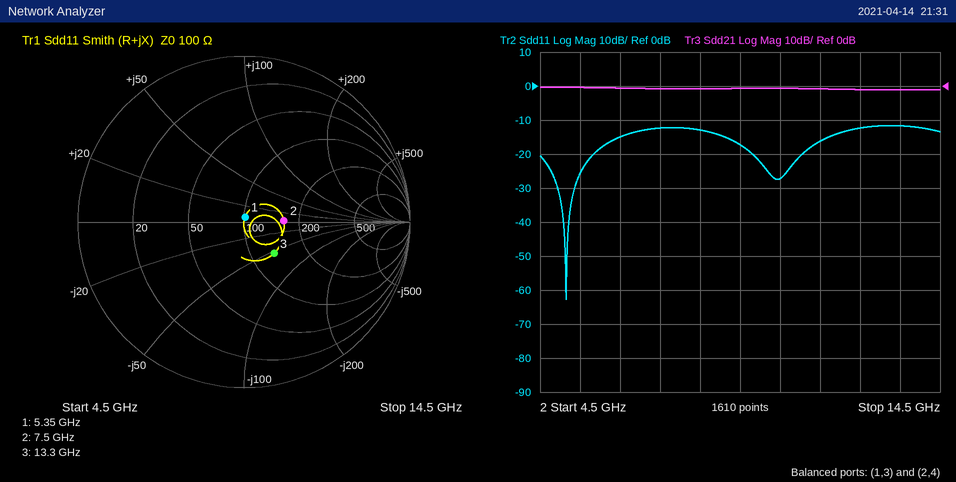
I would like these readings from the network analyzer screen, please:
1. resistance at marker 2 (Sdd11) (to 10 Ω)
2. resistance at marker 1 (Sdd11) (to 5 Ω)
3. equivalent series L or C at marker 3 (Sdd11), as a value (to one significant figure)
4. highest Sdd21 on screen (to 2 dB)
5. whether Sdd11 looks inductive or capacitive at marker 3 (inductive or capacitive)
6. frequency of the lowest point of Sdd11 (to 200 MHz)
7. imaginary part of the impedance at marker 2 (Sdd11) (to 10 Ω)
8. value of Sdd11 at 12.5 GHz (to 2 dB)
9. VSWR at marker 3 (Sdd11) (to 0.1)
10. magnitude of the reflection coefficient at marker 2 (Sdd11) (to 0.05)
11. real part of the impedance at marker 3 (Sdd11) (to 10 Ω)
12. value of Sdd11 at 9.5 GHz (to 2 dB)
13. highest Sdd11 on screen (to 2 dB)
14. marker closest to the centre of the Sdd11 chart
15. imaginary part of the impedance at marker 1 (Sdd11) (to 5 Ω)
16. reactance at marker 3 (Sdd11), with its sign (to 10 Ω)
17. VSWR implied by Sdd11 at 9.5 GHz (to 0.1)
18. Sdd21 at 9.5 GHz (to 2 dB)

160 Ω
100 Ω
200 fF
0 dB
capacitive
5.2 GHz
0 Ω
-12 dB
1.7
0.25
130 Ω
-18 dB
-12 dB
marker 1
+5 Ω
-50 Ω
1.3
0 dB
